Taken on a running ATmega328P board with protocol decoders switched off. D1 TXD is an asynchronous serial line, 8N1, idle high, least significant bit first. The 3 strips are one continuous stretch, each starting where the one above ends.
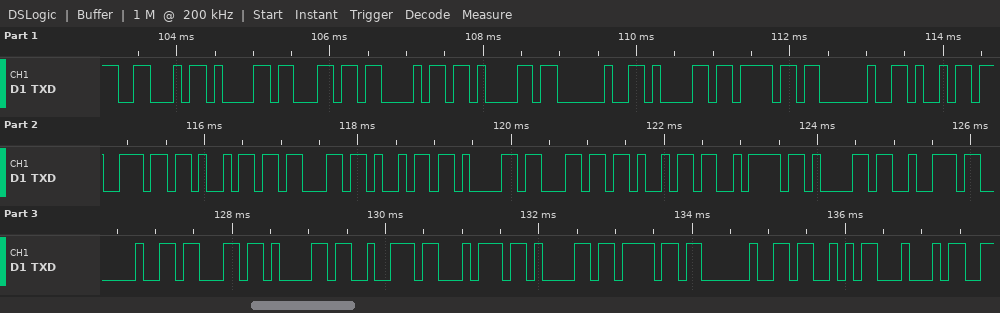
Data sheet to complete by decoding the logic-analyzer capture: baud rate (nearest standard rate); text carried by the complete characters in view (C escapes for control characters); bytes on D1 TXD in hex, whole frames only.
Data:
9600 baud
"Falha ao inicializar cartao SD"
46 61 6C 68 61 20 61 6F 20 69 6E 69 63 69 61 6C 69 7A 61 72 20 63 61 72 74 61 6F 20 53 44
